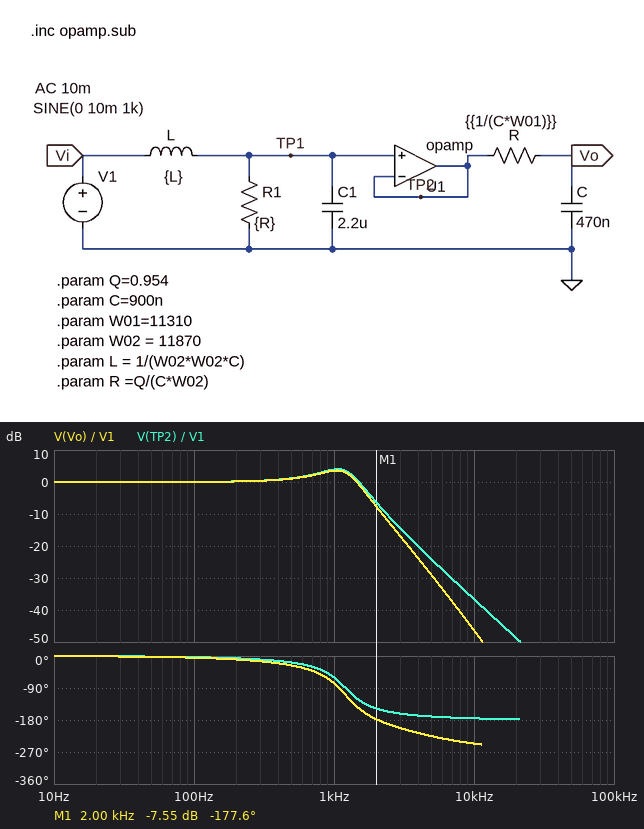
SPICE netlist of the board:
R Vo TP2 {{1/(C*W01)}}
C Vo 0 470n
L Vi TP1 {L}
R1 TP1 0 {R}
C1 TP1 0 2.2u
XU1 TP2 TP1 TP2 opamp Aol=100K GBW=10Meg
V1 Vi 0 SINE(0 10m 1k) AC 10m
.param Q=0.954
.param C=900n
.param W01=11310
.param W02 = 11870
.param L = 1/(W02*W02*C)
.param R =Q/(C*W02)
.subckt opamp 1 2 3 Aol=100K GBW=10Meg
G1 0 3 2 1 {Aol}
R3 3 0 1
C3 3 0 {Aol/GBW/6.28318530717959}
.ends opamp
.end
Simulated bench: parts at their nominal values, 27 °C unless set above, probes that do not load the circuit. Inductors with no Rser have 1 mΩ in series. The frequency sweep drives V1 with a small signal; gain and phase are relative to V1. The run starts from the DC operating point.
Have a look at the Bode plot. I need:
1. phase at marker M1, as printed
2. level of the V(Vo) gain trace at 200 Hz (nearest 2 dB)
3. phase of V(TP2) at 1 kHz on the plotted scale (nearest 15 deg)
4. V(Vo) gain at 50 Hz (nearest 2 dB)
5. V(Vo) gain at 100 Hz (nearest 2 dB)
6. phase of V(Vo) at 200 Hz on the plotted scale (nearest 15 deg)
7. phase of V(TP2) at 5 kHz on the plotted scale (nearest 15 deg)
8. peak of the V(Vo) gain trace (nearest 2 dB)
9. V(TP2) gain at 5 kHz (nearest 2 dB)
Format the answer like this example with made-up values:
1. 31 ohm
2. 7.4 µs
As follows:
1. -177.6 deg
2. 0 dB
3. -60 deg
4. 0 dB
5. 0 dB
6. -15 deg
7. -165 deg
8. 4 dB
9. -24 dB
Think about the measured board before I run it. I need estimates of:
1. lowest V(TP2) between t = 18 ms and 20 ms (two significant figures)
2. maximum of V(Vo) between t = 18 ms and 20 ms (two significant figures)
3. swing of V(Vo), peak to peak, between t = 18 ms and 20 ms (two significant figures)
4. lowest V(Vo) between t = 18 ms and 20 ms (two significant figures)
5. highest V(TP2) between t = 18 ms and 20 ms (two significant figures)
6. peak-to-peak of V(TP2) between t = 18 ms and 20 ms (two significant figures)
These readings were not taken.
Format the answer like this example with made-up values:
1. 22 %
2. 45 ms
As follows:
1. -16 mV
2. 15 mV
3. 30 mV
4. -15 mV
5. 16 mV
6. 31 mV
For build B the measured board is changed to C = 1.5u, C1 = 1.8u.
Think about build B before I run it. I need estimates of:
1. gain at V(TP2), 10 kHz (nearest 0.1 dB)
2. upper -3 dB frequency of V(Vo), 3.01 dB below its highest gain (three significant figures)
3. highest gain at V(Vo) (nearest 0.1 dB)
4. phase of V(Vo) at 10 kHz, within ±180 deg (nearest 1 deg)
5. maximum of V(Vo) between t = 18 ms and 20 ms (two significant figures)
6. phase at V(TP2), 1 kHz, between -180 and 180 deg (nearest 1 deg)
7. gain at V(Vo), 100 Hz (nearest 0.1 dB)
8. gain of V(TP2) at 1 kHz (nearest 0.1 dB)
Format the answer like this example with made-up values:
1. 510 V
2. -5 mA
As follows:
1. -34.9 dB
2. 1.44 kHz
3. 0.3 dB
4. 102 deg
5. 10 mV
6. -52 deg
7. 0 dB
8. 3.0 dB
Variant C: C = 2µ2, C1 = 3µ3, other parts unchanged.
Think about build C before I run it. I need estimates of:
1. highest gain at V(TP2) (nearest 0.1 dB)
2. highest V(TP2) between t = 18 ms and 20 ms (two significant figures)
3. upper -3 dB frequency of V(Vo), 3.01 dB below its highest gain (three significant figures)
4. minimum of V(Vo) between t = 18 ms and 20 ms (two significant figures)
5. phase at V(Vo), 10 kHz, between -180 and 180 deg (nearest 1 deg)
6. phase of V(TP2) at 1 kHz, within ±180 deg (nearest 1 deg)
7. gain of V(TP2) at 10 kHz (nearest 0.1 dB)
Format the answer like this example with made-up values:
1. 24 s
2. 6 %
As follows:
1. 5.6 dB
2. 18 mV
3. 1.09 kHz
4. -11 mV
5. 97 deg
6. -93 deg
7. -40.2 dB
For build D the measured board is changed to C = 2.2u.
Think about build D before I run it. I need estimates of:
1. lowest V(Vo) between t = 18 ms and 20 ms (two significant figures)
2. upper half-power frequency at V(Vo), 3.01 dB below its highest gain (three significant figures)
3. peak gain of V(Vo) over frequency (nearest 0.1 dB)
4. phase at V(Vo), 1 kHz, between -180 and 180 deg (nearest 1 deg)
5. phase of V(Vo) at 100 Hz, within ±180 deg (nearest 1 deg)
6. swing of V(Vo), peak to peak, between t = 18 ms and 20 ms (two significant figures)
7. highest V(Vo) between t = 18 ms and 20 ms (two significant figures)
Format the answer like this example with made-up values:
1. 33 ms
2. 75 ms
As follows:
1. -9.3 mV
2. 1.27 kHz
3. 0 dB
4. -114 deg
5. -11 deg
6. 19 mV
7. 9.3 mV
